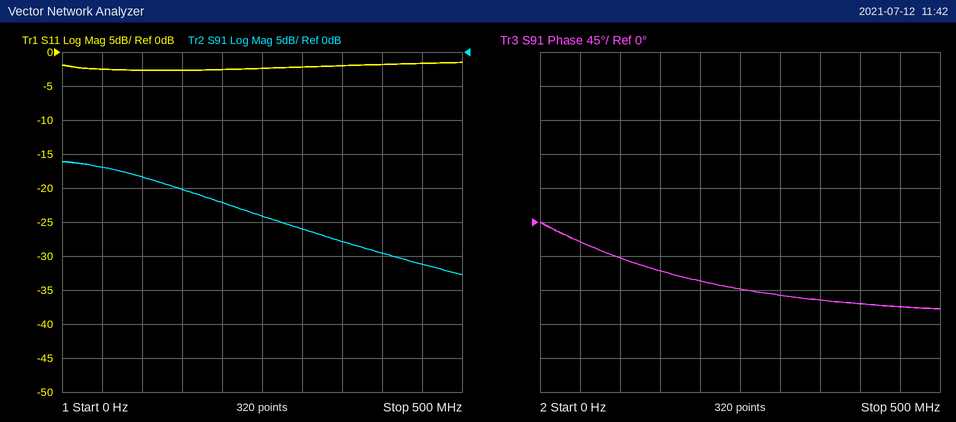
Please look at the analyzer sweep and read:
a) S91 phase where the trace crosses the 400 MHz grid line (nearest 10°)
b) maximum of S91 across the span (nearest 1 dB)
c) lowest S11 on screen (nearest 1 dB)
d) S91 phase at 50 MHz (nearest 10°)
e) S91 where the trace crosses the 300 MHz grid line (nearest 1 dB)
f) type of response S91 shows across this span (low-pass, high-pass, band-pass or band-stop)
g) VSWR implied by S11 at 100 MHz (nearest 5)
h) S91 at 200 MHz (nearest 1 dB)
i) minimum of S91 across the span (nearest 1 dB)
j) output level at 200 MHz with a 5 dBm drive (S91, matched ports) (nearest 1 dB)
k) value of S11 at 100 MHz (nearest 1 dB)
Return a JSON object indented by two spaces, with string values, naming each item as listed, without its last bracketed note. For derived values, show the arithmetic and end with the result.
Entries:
{
  "S91 phase where the trace crosses the 400 MHz grid line": "-110°",
  "maximum of S91 across the span": "-16 dB",
  "lowest S11 on screen": "-3 dB",
  "S91 phase at 50 MHz": "-30°",
  "S91 where the trace crosses the 300 MHz grid line": "-26 dB",
  "type of response S91 shows across this span": "low-pass",
  "VSWR implied by S11 at 100 MHz": "|Γ| = 10^(-3/20) = 0.7079; VSWR = (1 + 0.7079)/(1 − 0.7079) ≈ 5.85, so 5 to the nearest 5",
  "S91 at 200 MHz": "-22 dB",
  "minimum of S91 across the span": "-33 dB",
  "output level at 200 MHz with a 5 dBm drive (S91, matched ports)": "5 dBm + (-22 dB) = -17 dBm",
  "value of S11 at 100 MHz": "-3 dB"
}
